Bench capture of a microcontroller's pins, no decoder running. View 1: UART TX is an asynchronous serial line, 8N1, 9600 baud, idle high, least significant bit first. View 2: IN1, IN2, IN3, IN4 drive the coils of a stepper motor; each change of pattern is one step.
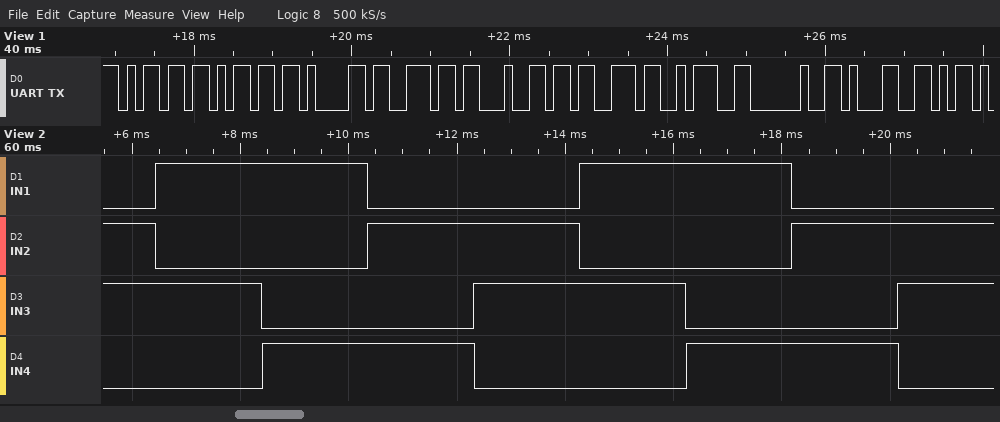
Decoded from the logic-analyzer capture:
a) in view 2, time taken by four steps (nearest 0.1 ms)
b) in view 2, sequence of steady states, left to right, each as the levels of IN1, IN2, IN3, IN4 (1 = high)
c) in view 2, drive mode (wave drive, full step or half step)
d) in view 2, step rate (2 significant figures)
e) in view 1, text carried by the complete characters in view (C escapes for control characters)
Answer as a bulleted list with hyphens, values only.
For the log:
- 7.8 ms
- 0110 1010 1001 0101 0110 1010 1001 0101 0110
- full step
- 510 steps/s
- "mmands: 1"
